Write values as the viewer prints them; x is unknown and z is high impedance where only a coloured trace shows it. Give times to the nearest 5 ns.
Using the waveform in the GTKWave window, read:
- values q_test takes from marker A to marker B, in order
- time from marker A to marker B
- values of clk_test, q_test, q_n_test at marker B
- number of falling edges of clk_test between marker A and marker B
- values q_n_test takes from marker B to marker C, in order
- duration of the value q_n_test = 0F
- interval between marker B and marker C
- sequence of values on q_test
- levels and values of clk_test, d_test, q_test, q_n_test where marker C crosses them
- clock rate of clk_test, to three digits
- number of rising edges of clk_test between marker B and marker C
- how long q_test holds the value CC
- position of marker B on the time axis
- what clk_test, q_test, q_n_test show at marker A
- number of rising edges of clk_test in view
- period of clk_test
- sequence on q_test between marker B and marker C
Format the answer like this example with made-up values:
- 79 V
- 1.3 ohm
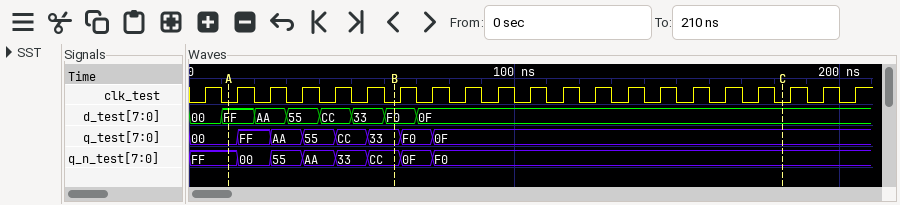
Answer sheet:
- 00, FF, AA, 55, CC, 33
- 50 ns
- clk_test=0, q_test=33, q_n_test=CC
- 5
- CC, 0F, F0
- 10 ns
- 120 ns
- 00, FF, AA, 55, CC, 33, F0, 0F
- clk_test=0, d_test=0F, q_test=0F, q_n_test=F0
- 100 MHz
- 12
- 10 ns
- 65 ns
- clk_test=0, q_test=00, q_n_test=FF
- 21
- 10 ns
- 33, F0, 0F
